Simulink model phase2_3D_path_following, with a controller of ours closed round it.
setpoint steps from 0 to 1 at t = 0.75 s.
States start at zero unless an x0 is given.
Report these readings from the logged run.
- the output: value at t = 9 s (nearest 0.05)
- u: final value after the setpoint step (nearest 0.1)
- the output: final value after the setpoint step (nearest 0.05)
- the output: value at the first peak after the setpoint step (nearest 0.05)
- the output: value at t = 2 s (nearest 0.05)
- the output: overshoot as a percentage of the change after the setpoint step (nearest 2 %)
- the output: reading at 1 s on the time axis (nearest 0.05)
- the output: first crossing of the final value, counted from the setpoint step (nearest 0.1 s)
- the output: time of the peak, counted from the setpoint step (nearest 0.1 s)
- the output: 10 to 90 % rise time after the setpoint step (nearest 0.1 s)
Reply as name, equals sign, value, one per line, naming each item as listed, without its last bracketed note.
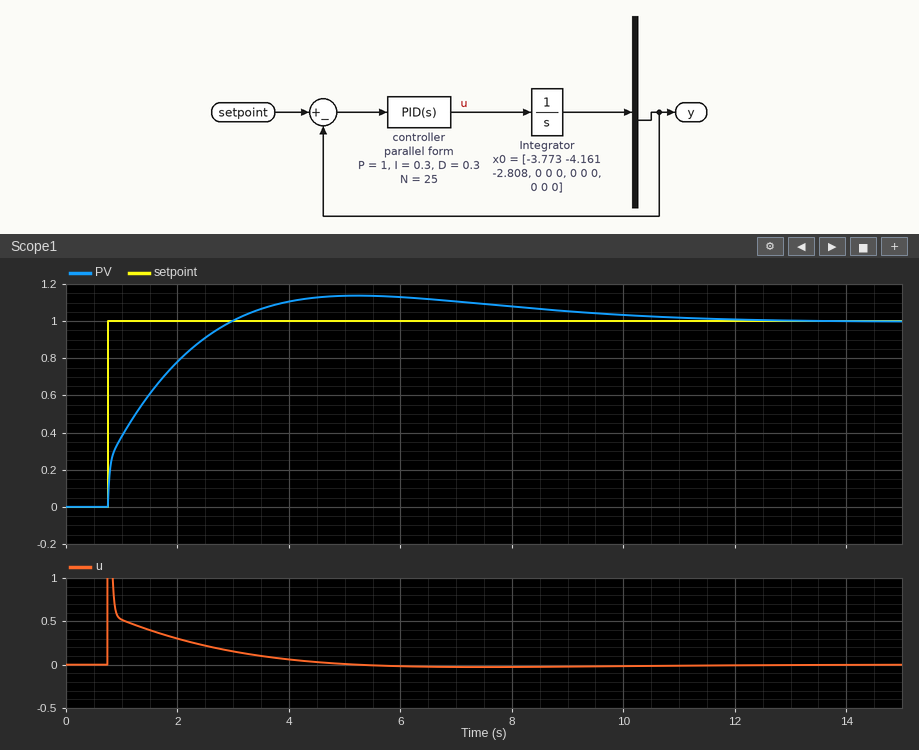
the output: value at t = 9 s = 1.05
u: final value after the setpoint step = 0.0
the output: final value after the setpoint step = 1.00
the output: value at the first peak after the setpoint step = 1.15
the output: value at t = 2 s = 0.80
the output: overshoot as a percentage of the change after the setpoint step = 14 %
the output: reading at 1 s on the time axis = 0.40
the output: first crossing of the final value, counted from the setpoint step = 2.2 s
the output: time of the peak, counted from the setpoint step = 4.5 s
the output: 10 to 90 % rise time after the setpoint step = 1.7 s
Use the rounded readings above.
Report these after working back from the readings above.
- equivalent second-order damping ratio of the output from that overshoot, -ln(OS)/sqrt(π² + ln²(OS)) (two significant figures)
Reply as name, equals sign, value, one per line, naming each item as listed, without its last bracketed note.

equivalent second-order damping ratio of the output from that overshoot, -ln(OS)/sqrt(π² + ln²(OS)) = 0.53
